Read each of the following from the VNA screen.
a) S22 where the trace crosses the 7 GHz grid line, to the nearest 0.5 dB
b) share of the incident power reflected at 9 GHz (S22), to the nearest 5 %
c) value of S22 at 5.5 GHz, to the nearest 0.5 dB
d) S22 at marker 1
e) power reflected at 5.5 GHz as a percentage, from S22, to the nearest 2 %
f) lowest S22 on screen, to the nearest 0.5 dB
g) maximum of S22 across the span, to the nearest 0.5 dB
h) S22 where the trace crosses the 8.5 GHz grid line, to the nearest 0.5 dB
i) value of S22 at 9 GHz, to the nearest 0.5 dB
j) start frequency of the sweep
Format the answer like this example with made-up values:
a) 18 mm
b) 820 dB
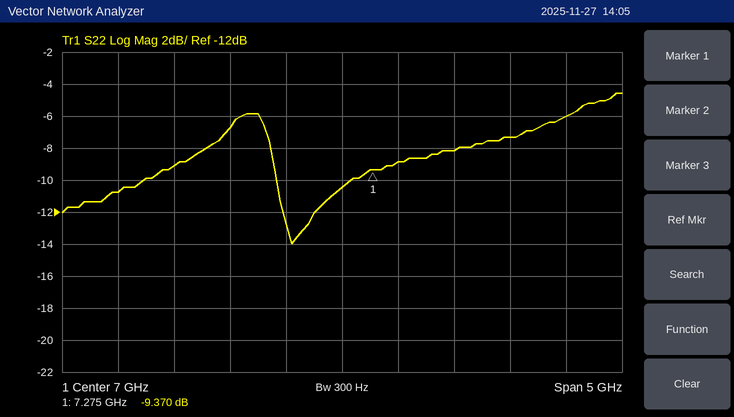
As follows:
a) -10.5 dB
b) 25 %
c) -9.0 dB
d) -9.370 dB
e) 12 %
f) -14.0 dB
g) -4.5 dB
h) -7.5 dB
i) -6.0 dB
j) 4.5 GHz
